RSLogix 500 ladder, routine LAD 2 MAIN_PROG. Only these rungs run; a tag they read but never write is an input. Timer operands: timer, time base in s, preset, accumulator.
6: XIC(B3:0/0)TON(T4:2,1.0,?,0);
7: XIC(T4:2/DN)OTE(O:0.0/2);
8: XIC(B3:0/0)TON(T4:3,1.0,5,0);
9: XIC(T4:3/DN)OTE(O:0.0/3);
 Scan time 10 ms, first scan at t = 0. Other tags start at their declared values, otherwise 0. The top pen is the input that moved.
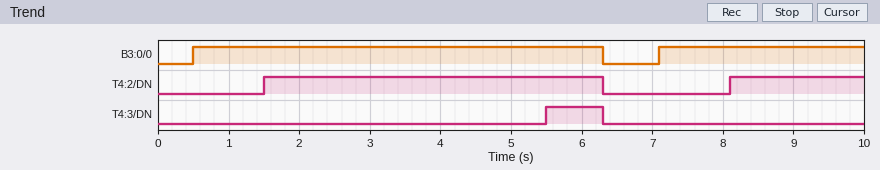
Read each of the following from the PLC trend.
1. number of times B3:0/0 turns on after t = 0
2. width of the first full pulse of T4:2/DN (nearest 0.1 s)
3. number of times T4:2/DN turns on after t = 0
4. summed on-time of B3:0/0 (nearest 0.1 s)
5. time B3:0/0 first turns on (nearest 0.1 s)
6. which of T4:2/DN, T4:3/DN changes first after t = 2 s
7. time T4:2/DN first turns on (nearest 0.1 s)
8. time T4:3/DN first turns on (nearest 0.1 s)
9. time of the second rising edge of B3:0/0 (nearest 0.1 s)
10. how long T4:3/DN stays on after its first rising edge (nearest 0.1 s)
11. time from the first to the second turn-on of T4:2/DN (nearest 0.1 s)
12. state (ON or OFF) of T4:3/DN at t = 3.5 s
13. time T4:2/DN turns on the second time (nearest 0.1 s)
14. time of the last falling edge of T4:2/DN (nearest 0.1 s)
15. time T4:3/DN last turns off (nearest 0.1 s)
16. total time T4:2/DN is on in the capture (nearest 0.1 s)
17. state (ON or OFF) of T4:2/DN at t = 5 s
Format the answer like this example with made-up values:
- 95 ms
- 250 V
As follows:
- 2
- 4.8 s
- 2
- 8.7 s
- 0.5 s
- T4:3/DN
- 1.5 s
- 5.5 s
- 7.1 s
- 0.8 s
- 6.6 s
- OFF
- 8.1 s
- 6.3 s
- 6.3 s
- 6.7 s
- ON
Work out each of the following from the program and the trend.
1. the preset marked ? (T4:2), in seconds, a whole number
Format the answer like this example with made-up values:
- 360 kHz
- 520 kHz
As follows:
- 1 s
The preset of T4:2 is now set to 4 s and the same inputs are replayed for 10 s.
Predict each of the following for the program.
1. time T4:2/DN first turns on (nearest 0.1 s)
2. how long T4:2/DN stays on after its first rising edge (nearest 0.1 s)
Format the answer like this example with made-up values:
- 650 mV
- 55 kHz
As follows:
- 4.5 s
- 1.8 s
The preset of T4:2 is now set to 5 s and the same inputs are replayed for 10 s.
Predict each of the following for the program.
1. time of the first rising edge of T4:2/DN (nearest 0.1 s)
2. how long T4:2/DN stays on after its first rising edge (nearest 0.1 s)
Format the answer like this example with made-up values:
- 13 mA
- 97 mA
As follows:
- 5.5 s
- 0.8 s
